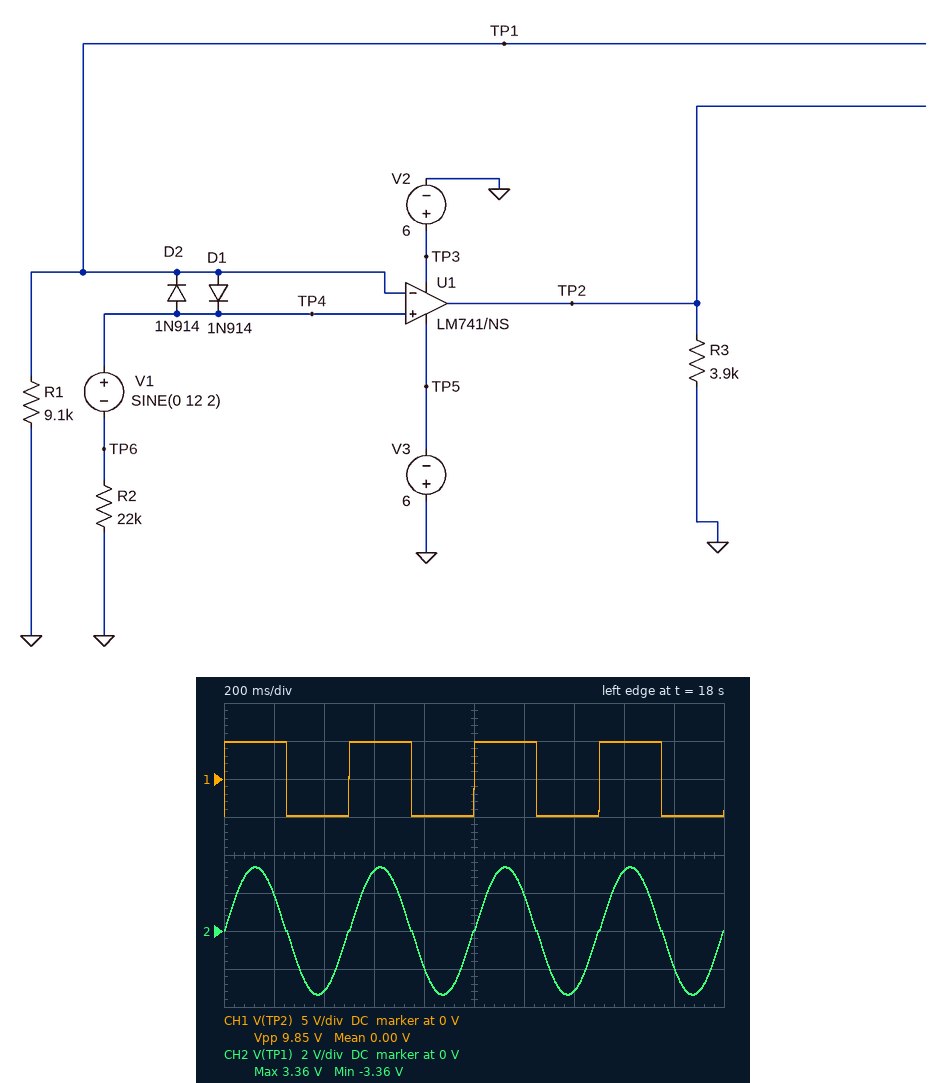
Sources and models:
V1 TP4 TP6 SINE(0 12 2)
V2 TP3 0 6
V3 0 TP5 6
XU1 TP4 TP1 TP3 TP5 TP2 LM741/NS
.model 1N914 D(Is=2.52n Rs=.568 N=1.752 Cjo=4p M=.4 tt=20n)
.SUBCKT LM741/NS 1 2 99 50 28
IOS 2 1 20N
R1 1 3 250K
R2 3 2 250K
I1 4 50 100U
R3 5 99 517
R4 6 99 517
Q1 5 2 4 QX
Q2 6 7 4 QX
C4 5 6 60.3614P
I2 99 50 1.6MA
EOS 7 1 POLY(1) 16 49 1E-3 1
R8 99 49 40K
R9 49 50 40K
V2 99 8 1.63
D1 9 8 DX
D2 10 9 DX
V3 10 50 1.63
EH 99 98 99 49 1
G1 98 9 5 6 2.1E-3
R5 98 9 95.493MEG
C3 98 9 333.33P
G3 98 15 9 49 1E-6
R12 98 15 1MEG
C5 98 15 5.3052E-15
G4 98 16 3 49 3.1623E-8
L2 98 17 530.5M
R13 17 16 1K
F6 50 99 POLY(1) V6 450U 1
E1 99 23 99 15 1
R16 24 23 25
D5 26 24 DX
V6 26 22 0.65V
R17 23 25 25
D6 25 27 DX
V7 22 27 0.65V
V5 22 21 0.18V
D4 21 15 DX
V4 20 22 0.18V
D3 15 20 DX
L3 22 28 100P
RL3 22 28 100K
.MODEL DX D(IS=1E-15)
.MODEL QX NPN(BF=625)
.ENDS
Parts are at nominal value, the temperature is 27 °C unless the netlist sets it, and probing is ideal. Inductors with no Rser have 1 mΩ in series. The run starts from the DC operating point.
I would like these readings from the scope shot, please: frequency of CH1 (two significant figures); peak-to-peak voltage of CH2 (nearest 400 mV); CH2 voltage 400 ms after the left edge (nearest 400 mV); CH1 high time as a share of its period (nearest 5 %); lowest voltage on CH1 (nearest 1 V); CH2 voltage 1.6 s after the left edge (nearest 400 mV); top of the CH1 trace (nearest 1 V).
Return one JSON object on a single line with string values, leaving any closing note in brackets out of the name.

{"frequency of CH1": "2.0 Hz", "peak-to-peak voltage of CH2": "6.8 V", "CH2 voltage 400 ms after the left edge": "-3.2 V", "CH1 high time as a share of its period": "50 %", "lowest voltage on CH1": "-5 V", "CH2 voltage 1.6 s after the left edge": "3.2 V", "top of the CH1 trace": "5 V"}
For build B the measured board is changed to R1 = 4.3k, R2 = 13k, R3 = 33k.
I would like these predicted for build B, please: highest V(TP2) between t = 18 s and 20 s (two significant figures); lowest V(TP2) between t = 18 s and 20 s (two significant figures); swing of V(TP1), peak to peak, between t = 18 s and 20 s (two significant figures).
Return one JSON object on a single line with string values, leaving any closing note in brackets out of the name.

{"highest V(TP2) between t = 18 s and 20 s": "5.0 V", "lowest V(TP2) between t = 18 s and 20 s": "-5.0 V", "swing of V(TP1), peak to peak, between t = 18 s and 20 s": "5.7 V"}
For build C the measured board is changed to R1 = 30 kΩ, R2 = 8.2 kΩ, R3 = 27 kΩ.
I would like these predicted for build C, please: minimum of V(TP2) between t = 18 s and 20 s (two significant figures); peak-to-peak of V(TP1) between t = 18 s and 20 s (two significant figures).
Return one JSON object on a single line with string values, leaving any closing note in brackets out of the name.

{"minimum of V(TP2) between t = 18 s and 20 s": "-5.0 V", "peak-to-peak of V(TP1) between t = 18 s and 20 s": "15 V"}
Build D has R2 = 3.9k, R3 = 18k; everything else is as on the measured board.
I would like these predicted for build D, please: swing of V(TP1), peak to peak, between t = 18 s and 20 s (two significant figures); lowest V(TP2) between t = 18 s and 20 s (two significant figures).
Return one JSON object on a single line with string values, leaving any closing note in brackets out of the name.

{"swing of V(TP1), peak to peak, between t = 18 s and 20 s": "14 V", "lowest V(TP2) between t = 18 s and 20 s": "-5.0 V"}
